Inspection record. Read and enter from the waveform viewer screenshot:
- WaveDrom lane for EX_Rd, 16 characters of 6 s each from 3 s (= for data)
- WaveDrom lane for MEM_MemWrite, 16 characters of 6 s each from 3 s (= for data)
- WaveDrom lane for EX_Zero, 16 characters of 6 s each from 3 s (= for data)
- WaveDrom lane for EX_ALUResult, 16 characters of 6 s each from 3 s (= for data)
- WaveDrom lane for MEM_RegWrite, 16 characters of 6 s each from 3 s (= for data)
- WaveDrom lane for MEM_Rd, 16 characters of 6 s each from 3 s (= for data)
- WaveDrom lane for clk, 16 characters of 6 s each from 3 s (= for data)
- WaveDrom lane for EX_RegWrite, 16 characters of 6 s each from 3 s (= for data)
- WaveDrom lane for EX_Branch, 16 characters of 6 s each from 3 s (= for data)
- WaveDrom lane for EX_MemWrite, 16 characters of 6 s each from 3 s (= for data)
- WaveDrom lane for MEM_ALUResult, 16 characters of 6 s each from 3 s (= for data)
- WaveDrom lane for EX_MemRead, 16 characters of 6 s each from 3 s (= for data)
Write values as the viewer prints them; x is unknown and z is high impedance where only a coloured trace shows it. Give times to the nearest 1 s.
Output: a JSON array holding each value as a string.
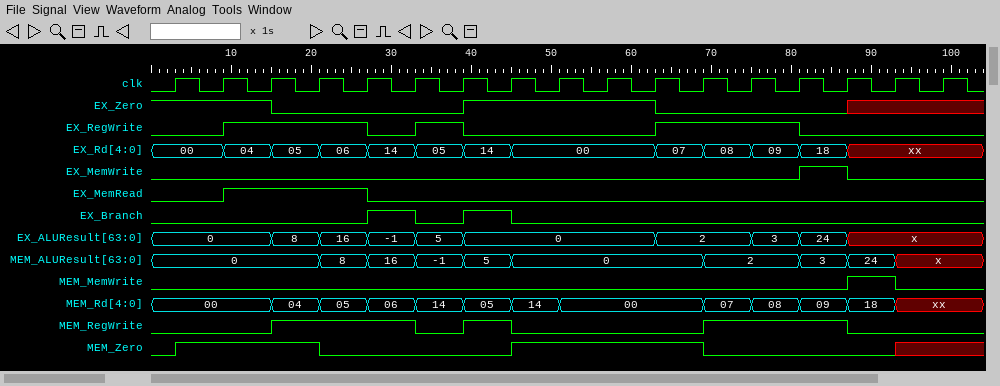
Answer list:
["{name: 'EX_Rd', wave: '========..====x.', data: '00 04 05 06 14 05 14 00 07 08 09 18'}", "{name: 'MEM_MemWrite', wave: '0.............10'}", "{name: 'EX_Zero', wave: '1.0...1...0...x.'}", "{name: 'EX_ALUResult', wave: '=.=====...=.==x.', data: '0 8 16 -1 5 0 2 3 24'}", "{name: 'MEM_RegWrite', wave: '0.1..010...1..0.'}", "{name: 'MEM_Rd', wave: '=.=======..====x', data: '00 04 05 06 14 05 14 00 07 08 09 18'}", "{name: 'clk', wave: 'p...............'}", "{name: 'EX_RegWrite', wave: '01..010...1..0..'}", "{name: 'EX_Branch', wave: '0...1010........'}", "{name: 'EX_MemWrite', wave: '0............10.'}", "{name: 'MEM_ALUResult', wave: '=..=====...=.==x', data: '0 8 16 -1 5 0 2 3 24'}", "{name: 'EX_MemRead', wave: '01..0...........'}"]
